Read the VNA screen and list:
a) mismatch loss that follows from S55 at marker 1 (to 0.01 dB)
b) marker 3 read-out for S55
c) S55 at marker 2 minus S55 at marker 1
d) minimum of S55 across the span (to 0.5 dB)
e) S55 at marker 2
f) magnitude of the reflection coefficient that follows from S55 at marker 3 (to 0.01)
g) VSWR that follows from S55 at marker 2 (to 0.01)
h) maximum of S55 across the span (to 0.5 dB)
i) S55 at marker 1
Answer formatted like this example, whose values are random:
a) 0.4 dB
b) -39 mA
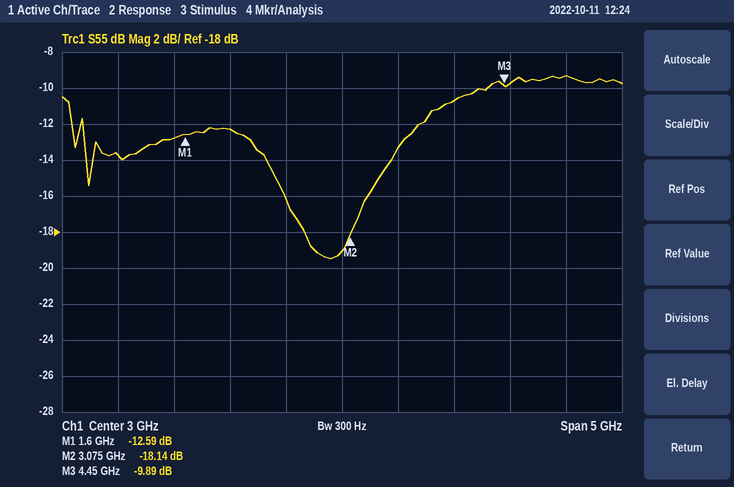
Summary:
a) 0.25 dB
b) -9.89 dB
c) -5.55 dB
d) -19.5 dB
e) -18.14 dB
f) 0.32
g) 1.28
h) -9.5 dB
i) -12.59 dB
